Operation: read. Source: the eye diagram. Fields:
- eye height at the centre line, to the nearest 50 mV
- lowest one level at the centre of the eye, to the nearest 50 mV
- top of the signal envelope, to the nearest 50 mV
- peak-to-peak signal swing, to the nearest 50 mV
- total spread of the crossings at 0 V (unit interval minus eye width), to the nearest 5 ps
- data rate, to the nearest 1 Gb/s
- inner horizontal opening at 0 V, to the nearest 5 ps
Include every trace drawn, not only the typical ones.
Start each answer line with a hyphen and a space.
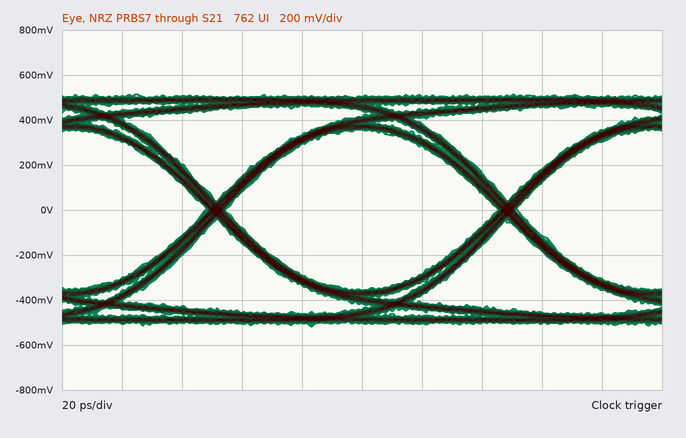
- 700 mV
- 350 mV
- 500 mV
- 1.05 V
- 5 ps
- 10 Gb/s
- 90 ps
